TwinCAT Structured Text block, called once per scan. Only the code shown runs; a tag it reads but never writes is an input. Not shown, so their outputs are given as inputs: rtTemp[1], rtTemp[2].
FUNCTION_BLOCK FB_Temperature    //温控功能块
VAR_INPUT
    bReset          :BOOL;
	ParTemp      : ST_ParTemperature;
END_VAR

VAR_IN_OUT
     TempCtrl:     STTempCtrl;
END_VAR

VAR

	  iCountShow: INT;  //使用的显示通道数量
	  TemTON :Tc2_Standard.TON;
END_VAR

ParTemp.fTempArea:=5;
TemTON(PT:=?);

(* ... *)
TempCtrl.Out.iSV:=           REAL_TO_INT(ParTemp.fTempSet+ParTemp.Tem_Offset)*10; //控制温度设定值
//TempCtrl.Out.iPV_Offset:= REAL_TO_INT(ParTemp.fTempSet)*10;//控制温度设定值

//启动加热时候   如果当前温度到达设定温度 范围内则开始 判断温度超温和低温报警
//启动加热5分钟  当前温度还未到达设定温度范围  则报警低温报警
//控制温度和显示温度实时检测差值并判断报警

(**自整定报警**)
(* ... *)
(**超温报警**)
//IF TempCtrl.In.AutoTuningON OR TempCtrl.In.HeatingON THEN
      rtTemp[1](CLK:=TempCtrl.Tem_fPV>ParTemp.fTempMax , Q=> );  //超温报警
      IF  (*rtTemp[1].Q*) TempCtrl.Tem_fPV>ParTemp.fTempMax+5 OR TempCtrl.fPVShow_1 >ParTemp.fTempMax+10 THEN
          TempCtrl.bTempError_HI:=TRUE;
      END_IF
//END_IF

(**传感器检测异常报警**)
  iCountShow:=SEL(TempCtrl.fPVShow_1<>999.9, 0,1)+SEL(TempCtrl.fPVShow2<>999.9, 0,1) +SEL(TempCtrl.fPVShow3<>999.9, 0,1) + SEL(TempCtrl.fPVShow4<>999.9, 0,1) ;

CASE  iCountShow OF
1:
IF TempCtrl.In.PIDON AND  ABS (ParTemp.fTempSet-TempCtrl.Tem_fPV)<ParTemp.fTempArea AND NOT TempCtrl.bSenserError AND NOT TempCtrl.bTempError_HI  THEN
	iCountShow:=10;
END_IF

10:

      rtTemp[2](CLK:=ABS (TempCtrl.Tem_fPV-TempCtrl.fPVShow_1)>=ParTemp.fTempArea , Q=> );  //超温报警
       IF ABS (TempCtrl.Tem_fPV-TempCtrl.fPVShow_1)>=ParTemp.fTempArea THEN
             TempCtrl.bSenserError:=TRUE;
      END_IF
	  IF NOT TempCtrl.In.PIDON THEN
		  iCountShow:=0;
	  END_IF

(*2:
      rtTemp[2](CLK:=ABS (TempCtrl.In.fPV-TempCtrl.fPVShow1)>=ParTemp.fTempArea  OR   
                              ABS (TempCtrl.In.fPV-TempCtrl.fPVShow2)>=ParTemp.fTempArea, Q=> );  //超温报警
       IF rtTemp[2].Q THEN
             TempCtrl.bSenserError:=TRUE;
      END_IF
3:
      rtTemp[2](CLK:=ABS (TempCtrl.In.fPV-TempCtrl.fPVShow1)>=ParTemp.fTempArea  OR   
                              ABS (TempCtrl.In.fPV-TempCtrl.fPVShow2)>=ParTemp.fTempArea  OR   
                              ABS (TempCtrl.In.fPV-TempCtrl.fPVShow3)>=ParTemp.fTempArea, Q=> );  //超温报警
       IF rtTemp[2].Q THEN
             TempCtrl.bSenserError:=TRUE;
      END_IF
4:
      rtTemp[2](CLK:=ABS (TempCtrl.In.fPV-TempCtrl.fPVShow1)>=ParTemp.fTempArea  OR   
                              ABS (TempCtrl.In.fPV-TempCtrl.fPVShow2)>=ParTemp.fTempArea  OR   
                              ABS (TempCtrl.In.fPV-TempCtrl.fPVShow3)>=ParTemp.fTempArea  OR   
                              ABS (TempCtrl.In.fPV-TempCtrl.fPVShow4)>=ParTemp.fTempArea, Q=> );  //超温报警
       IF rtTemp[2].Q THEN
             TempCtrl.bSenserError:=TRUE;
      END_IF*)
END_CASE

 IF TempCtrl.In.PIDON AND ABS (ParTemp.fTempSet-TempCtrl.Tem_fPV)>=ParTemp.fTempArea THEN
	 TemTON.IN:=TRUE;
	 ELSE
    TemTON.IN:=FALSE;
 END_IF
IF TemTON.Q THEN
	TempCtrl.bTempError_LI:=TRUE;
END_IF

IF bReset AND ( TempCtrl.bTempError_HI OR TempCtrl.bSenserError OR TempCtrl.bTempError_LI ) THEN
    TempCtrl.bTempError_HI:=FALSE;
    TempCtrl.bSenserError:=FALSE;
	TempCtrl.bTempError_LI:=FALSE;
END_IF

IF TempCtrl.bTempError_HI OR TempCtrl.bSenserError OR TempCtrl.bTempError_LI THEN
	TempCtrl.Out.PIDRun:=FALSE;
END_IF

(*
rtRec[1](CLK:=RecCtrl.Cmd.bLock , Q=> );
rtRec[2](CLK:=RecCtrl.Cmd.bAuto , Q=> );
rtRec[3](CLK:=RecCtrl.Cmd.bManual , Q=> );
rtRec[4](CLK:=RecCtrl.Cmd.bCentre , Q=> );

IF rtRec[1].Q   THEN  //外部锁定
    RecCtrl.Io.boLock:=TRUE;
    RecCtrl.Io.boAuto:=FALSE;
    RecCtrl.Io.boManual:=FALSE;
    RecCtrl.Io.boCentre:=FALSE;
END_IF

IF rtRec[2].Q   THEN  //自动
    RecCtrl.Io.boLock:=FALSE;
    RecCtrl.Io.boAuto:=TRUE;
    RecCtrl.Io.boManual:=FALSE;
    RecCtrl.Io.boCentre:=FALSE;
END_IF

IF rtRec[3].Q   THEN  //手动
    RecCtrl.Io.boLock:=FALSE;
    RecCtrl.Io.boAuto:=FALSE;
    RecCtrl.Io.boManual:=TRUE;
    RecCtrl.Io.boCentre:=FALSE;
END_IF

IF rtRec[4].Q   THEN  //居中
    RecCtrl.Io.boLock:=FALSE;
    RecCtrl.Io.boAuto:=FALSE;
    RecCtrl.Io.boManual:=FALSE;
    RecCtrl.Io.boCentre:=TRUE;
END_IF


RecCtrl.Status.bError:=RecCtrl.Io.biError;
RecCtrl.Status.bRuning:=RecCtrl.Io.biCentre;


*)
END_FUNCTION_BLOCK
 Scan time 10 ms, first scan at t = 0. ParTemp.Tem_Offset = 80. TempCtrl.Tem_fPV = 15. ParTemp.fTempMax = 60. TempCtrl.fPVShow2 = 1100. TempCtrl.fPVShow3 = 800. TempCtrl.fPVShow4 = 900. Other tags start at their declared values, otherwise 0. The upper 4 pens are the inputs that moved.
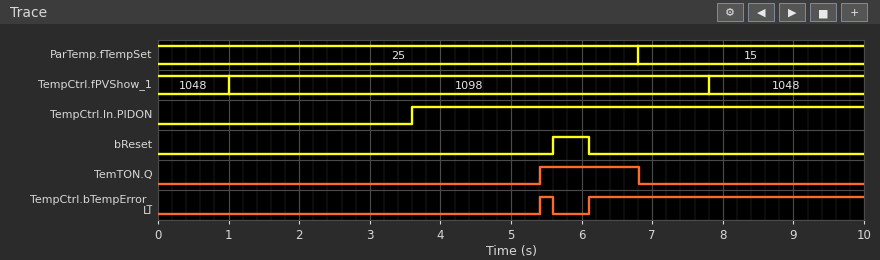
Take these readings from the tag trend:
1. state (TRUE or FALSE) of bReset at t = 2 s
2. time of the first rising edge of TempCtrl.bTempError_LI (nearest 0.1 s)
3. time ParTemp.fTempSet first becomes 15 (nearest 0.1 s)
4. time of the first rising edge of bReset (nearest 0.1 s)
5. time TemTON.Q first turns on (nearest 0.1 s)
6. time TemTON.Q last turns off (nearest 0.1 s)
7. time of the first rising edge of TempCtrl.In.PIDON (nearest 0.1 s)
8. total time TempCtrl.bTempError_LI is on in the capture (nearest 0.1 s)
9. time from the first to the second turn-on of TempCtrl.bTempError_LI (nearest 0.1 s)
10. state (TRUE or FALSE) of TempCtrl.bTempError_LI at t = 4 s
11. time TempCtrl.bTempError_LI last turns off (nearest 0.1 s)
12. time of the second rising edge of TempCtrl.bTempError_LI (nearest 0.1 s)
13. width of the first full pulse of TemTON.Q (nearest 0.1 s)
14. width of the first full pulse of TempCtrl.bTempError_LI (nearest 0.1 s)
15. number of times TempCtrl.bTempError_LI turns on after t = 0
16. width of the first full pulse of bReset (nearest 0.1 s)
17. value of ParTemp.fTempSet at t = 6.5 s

FALSE
5.4 s
6.8 s
5.6 s
5.4 s
6.8 s
3.6 s
4.1 s
0.7 s
FALSE
5.6 s
6.1 s
1.4 s
0.2 s
2
0.5 s
25
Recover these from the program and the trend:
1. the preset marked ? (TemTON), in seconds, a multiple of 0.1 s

1.8 s
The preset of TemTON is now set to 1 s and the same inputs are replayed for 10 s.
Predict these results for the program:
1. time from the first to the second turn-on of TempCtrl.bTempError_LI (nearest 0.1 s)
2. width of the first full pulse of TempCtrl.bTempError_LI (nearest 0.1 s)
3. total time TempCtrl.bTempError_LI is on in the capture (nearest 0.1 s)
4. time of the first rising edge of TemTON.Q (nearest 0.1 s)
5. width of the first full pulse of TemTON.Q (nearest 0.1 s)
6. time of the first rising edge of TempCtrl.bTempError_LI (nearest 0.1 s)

1.5 s
1.0 s
4.9 s
4.6 s
2.2 s
4.6 s
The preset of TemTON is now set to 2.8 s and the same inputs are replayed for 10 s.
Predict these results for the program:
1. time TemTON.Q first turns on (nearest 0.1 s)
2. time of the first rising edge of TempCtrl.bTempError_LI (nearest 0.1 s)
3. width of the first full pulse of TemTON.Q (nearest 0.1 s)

6.4 s
6.4 s
0.4 s
